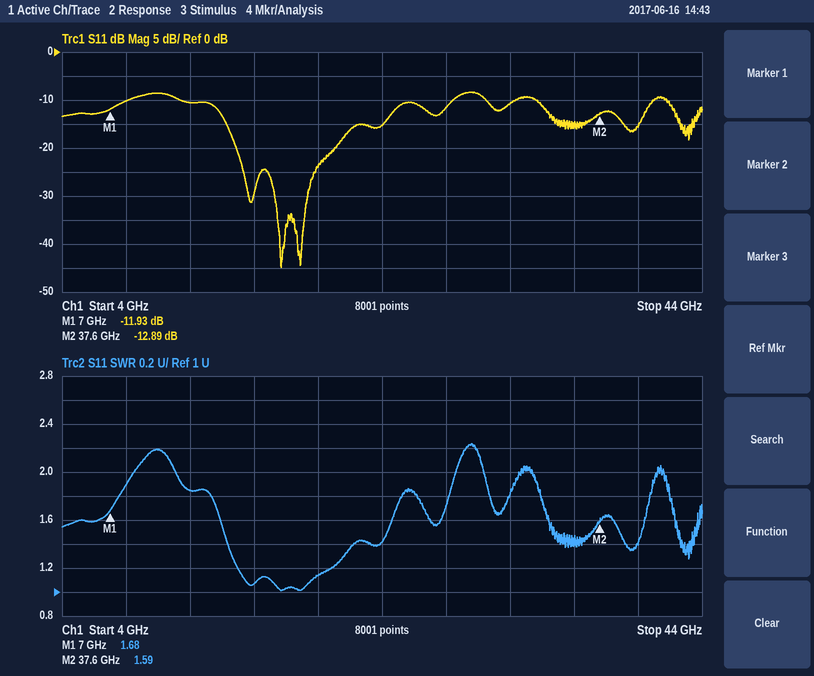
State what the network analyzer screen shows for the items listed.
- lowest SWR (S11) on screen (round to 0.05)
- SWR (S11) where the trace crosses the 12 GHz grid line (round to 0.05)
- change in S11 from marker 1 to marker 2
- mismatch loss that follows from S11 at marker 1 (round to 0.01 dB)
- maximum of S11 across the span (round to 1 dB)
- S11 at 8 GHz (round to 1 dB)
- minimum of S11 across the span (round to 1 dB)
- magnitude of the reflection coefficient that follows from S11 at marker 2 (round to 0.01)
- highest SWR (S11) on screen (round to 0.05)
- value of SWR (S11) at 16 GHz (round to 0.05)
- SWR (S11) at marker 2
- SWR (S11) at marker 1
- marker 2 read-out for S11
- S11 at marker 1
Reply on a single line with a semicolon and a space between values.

1.00; 1.85; -0.96 dB; 0.29 dB; -8 dB; -10 dB; -45 dB; 0.23; 2.25; 1.05; 1.59; 1.68; -12.89 dB; -11.93 dB
